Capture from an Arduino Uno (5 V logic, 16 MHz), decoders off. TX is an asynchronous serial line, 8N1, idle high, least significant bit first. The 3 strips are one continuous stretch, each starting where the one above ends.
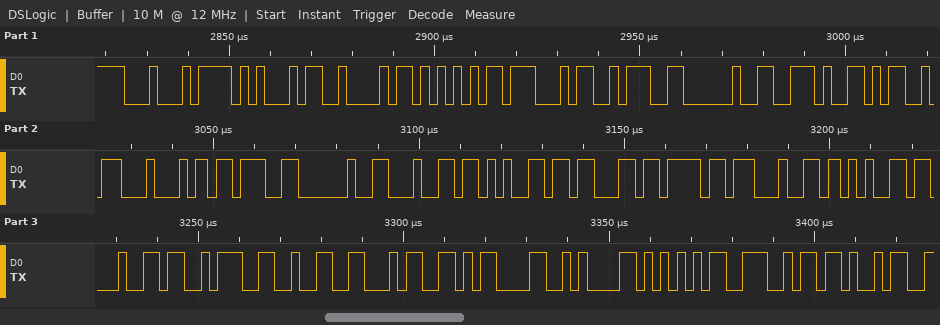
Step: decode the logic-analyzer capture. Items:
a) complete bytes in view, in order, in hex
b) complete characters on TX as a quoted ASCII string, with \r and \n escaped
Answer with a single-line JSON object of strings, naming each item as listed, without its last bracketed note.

{"complete bytes in view, in order, in hex": "0x44 0x45 0x42 0x55 0x47 0x3A 0x20 0x2E 0x4D 0x44 0x3B 0x20 0x64 0x65 0x63 0x6F 0x64 0x65 0x64 0x3A 0x32 0x34 0x0D 0x0A 0x55 0x4E 0x4B", "complete characters on TX as a quoted ASCII string, with \\r and \\n escaped": "\"DEBUG: .MD; decoded:24\\r\\nUNK\""}
